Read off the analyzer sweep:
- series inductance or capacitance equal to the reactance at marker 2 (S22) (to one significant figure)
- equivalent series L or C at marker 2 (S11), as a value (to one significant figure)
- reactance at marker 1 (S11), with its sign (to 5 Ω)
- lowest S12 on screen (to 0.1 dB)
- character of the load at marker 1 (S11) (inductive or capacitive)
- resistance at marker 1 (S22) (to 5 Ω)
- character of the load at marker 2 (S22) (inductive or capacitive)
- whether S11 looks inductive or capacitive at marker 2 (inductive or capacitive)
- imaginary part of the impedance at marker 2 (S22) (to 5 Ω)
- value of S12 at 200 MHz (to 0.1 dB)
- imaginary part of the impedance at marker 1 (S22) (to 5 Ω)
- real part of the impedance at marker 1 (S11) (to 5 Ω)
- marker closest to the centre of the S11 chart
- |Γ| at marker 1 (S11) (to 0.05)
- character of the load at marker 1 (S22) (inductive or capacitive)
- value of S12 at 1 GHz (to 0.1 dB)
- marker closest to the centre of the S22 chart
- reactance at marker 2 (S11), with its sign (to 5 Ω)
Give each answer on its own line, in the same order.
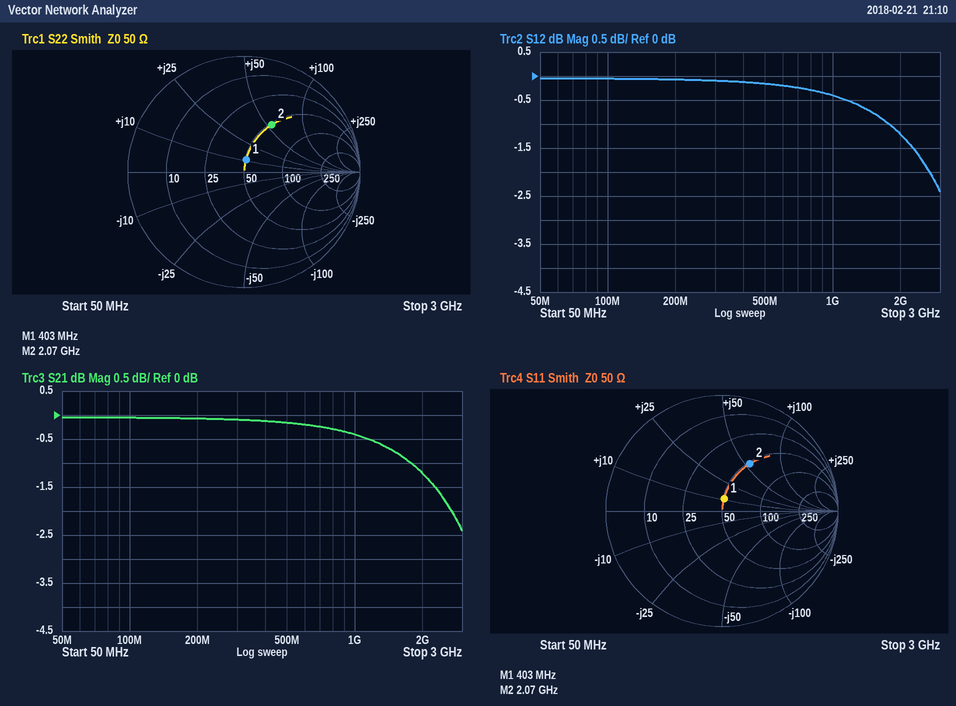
4 nH
4 nH
+10 Ω
-2.4 dB
inductive
50 Ω
inductive
inductive
+55 Ω
-0.1 dB
+10 Ω
50 Ω
marker 1
0.10
inductive
-0.4 dB
marker 1
+55 Ω
